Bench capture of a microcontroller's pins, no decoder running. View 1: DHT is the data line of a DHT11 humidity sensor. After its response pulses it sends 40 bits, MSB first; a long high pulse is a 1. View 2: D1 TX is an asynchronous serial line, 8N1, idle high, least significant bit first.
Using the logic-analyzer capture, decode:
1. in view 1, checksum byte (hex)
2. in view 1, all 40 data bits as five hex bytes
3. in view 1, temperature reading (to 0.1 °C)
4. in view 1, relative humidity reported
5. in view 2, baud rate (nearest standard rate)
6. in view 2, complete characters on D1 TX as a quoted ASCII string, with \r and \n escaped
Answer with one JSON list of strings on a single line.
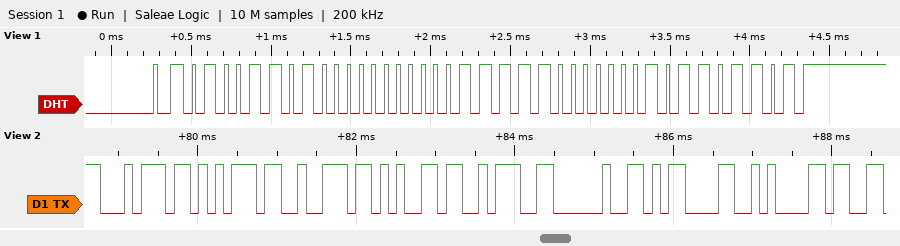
["0x6D", "4D 00 1F 01 6D", "31.1 °C", "77 %", "9600 baud", "\"ture: \\r\\n\""]
